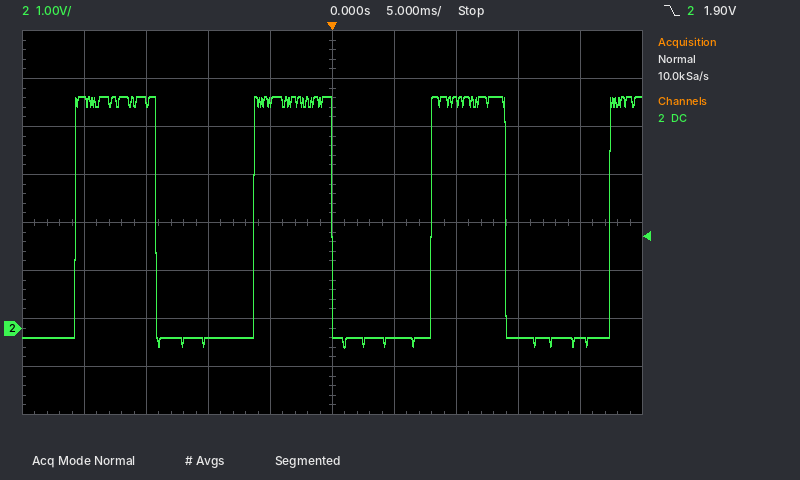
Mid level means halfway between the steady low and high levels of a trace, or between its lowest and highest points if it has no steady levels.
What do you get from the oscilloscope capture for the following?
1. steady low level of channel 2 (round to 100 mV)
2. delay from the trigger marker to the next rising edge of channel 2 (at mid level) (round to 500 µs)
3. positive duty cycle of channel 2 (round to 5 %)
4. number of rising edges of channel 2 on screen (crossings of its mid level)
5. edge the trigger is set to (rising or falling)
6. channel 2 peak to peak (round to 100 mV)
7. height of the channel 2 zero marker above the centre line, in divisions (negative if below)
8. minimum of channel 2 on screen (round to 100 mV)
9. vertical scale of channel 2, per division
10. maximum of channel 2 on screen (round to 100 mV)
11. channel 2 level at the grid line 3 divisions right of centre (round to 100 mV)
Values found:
-200 mV
8.0 ms
45 %
4
falling
5.2 V
-2.2 div
-400 mV
1 V
4.8 V
-200 mV
